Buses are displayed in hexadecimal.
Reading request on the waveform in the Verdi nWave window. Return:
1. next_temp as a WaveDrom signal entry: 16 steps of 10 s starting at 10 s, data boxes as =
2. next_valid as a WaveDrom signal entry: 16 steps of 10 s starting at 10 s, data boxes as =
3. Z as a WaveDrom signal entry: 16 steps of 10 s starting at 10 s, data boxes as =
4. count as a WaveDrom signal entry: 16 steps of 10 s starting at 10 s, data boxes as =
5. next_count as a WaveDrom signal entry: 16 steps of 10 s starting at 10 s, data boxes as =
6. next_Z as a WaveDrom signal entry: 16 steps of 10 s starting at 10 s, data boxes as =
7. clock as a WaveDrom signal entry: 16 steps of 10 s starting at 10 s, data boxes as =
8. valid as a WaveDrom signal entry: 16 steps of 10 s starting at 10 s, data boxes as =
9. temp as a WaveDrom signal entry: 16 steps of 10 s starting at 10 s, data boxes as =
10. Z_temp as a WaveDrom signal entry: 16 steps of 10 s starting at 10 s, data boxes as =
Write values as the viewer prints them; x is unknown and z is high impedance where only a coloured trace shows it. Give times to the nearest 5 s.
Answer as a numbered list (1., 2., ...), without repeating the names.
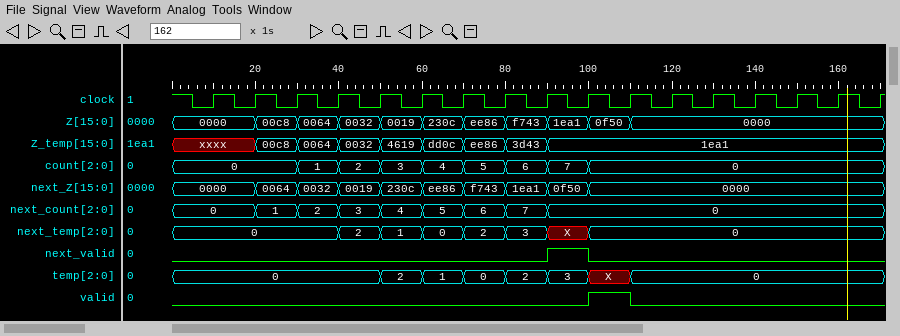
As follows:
1. {name: 'next_temp', wave: '=..=======......', data: '0 2 1 0 2 3 X 0'}
2. {name: 'next_valid', wave: '0.......10......'}
3. {name: 'Z', wave: '===========.....', data: '0000 00c8 0064 0032 0019 230c ee86 f743 1ea1 0f50 0000'}
4. {name: 'count', wave: '=.========......', data: '0 1 2 3 4 5 6 7 0'}
5. {name: 'next_count', wave: '=========.......', data: '0 1 2 3 4 5 6 7 0'}
6. {name: 'next_Z', wave: '==========......', data: '0000 0064 0032 0019 230c ee86 f743 1ea1 0f50 0000'}
7. {name: 'clock', wave: 'p...............'}
8. {name: 'valid', wave: '0........10.....'}
9. {name: 'temp', wave: '=...=======.....', data: '0 2 1 0 2 3 X 0'}
10. {name: 'Z_temp', wave: 'x========.......', data: '00c8 0064 0032 4619 dd0c ee86 3d43 1ea1'}
